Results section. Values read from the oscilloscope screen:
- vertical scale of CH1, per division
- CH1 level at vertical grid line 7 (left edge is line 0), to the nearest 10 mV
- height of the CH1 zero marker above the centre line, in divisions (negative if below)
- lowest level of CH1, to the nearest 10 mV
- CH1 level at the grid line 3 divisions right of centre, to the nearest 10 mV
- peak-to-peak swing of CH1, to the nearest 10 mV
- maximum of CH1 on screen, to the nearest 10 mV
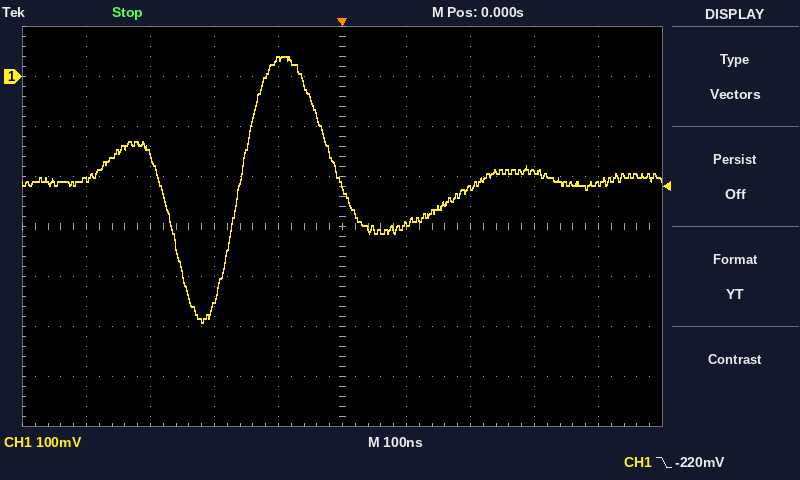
100 mV
-220 mV
+3.0 div
-490 mV
-190 mV
530 mV
40 mV
